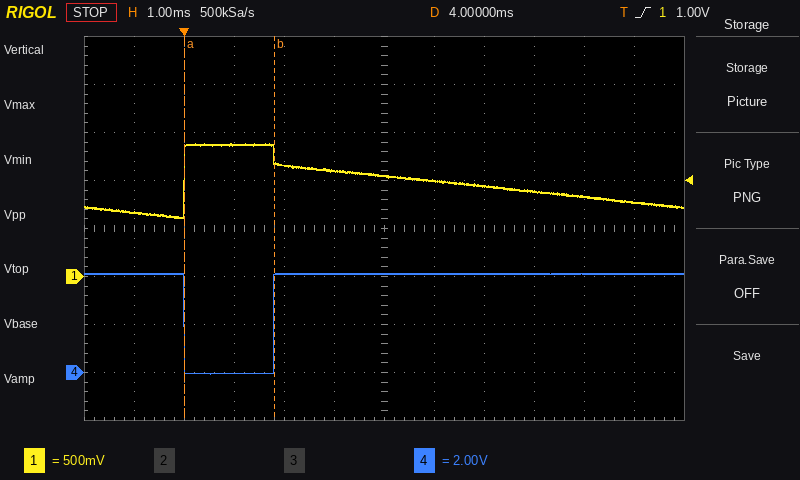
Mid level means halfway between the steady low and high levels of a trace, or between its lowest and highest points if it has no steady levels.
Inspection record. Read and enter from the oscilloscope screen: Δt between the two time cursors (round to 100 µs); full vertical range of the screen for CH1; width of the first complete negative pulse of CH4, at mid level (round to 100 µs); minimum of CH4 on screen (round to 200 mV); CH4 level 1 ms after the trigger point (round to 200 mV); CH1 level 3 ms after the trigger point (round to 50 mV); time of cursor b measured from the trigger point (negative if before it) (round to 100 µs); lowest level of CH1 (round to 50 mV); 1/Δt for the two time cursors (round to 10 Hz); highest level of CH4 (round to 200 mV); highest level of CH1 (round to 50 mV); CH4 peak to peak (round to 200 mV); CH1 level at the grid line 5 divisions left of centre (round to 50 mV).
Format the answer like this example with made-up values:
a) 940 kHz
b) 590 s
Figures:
a) 1.8 ms
b) 4 V
c) 1.8 ms
d) 0.0 V
e) 0.0 V
f) 1.10 V
g) +1.8 ms
h) 600 mV
i) 560 Hz
j) 4.2 V
k) 1.40 V
l) 4.2 V
m) 650 mV
